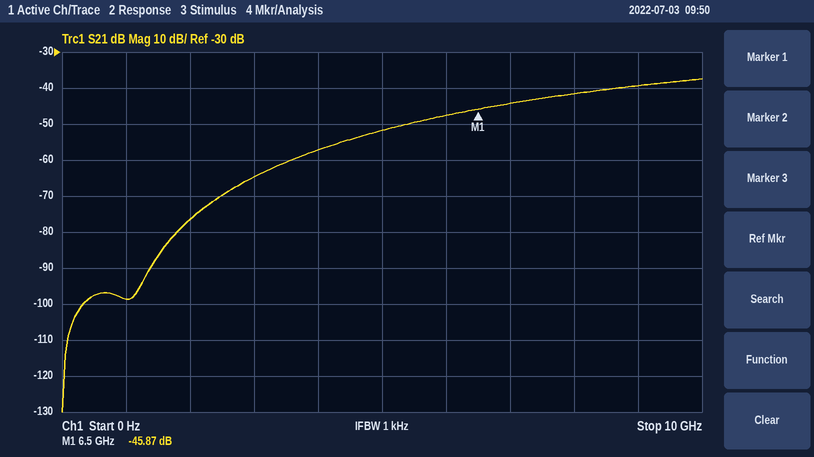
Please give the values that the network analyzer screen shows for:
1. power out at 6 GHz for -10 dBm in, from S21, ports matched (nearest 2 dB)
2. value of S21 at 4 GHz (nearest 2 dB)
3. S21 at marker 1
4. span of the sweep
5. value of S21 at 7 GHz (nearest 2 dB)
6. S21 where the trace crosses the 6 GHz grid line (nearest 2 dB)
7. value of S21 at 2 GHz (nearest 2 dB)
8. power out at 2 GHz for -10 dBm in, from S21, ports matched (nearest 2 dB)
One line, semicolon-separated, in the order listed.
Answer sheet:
-58 dBm; -58 dB; -45.87 dB; 10 GHz; -44 dB; -48 dB; -76 dB; -86 dBm
